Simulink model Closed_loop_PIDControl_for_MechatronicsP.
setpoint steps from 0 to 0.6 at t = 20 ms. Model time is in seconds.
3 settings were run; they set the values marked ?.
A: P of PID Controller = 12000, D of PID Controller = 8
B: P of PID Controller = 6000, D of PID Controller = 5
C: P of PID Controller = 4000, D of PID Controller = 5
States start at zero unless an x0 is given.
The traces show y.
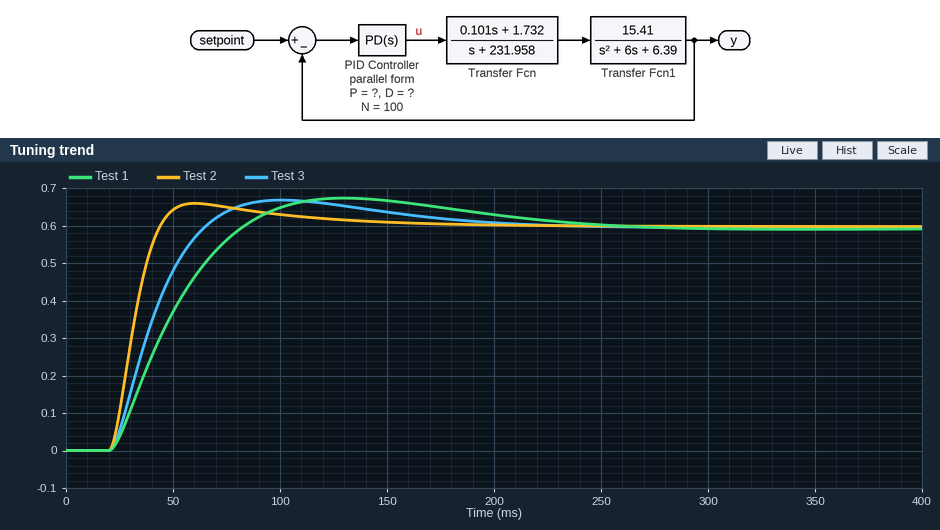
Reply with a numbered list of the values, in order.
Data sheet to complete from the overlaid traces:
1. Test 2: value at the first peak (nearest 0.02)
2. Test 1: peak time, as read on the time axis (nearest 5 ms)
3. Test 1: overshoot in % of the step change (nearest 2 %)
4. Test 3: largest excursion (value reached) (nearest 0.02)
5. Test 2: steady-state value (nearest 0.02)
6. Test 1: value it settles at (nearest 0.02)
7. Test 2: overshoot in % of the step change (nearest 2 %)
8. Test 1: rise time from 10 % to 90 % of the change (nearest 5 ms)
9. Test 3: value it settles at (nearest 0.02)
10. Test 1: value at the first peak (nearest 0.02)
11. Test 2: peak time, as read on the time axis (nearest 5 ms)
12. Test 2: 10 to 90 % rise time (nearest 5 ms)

1. 0.66
2. 130 ms
3. 14 %
4. 0.66
5. 0.60
6. 0.60
7. 10 %
8. 45 ms
9. 0.60
10. 0.68
11. 60 ms
12. 15 ms
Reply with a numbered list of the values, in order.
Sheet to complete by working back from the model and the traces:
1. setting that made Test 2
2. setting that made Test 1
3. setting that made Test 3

1. A
2. C
3. B
